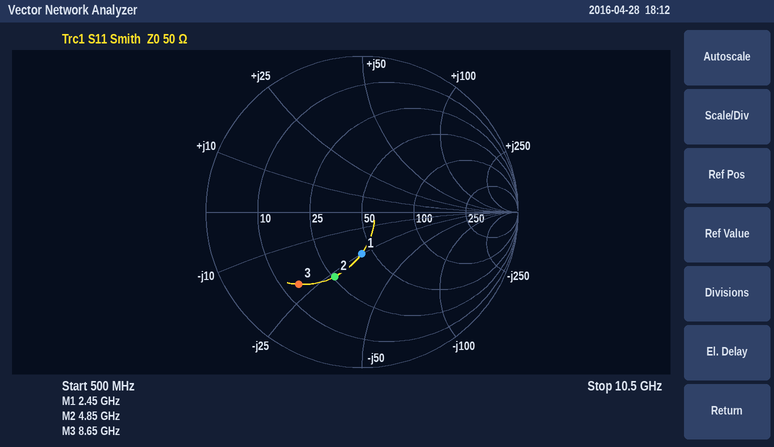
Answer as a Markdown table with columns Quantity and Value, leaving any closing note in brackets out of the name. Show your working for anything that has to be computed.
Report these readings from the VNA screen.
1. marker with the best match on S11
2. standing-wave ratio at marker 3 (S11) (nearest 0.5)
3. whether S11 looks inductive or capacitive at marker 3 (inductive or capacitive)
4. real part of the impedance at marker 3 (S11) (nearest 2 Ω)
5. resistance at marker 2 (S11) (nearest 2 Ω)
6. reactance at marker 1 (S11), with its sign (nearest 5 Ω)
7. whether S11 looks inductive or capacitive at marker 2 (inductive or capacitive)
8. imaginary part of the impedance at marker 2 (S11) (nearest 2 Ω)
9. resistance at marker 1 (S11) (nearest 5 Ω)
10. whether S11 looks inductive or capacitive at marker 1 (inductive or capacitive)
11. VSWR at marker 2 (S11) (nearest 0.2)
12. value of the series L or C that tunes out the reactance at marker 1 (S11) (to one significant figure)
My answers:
| Quantity | Value |
|---|---|
| marker with the best match on S11 | marker 1 |
| standing-wave ratio at marker 3 (S11) | 4.0 |
| whether S11 looks inductive or capacitive at marker 3 | capacitive |
| real part of the impedance at marker 3 (S11) | 14 Ω |
| resistance at marker 2 (S11) | 26 Ω |
| reactance at marker 1 (S11), with its sign | -25 Ω |
| whether S11 looks inductive or capacitive at marker 2 | capacitive |
| imaginary part of the impedance at marker 2 (S11) | -26 Ω |
| resistance at marker 1 (S11) | 45 Ω |
| whether S11 looks inductive or capacitive at marker 1 | capacitive |
| VSWR at marker 2 (S11) | 2.6 |
| value of the series L or C that tunes out the reactance at marker 1 (S11) | L = 25 Ω/(2π × 2.45 GHz) ≈ 2 nH |
